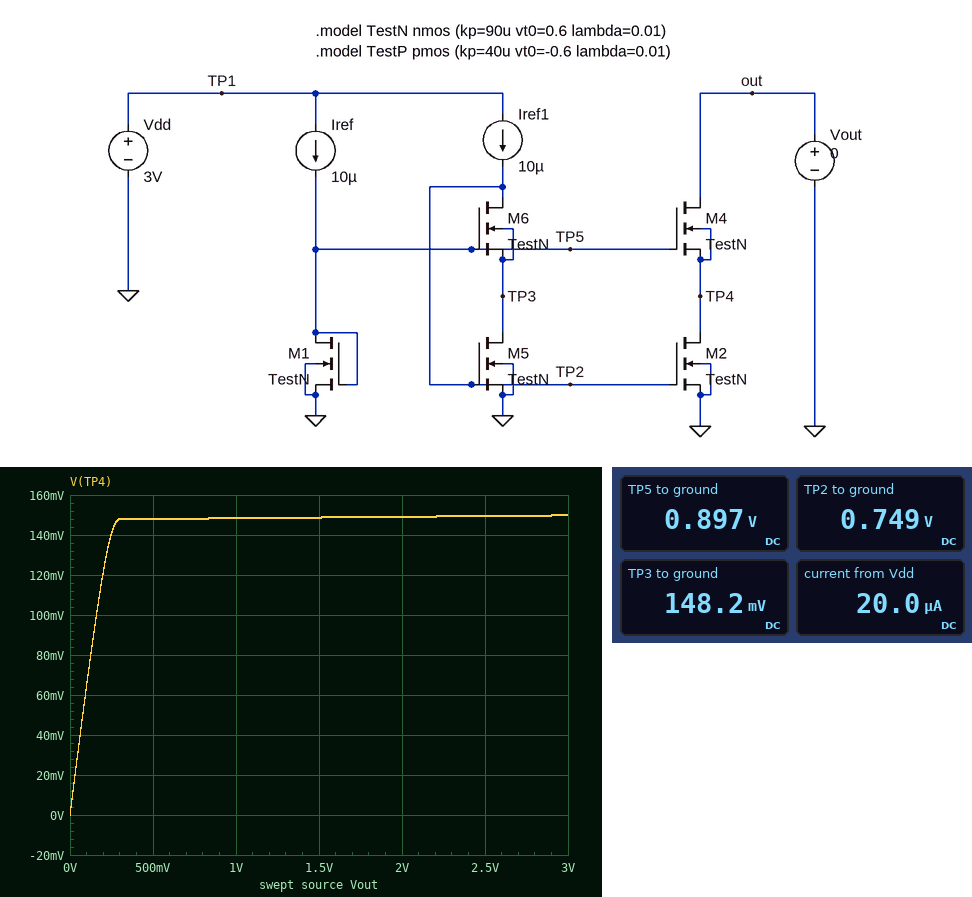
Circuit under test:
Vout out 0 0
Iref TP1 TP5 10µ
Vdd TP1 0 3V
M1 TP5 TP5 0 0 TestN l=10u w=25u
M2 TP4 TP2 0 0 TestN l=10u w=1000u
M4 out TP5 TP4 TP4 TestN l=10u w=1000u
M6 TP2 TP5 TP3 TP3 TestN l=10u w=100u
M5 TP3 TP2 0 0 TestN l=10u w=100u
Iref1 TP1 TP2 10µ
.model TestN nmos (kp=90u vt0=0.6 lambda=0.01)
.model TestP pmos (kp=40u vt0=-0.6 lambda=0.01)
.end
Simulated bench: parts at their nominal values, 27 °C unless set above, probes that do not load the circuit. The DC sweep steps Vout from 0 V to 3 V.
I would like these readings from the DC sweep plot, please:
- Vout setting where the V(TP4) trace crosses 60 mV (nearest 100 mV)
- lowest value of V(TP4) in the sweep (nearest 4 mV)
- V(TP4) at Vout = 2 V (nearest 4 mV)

100 mV
0 V
148 mV
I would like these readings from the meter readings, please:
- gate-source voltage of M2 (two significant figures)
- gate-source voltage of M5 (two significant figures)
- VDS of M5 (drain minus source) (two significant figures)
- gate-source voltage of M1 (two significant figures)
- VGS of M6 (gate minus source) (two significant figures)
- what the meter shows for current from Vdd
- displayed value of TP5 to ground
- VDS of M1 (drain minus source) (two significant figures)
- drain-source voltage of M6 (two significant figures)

750 mV
750 mV
150 mV
900 mV
750 mV
20.0 µA
0.897 V
900 mV
600 mV
